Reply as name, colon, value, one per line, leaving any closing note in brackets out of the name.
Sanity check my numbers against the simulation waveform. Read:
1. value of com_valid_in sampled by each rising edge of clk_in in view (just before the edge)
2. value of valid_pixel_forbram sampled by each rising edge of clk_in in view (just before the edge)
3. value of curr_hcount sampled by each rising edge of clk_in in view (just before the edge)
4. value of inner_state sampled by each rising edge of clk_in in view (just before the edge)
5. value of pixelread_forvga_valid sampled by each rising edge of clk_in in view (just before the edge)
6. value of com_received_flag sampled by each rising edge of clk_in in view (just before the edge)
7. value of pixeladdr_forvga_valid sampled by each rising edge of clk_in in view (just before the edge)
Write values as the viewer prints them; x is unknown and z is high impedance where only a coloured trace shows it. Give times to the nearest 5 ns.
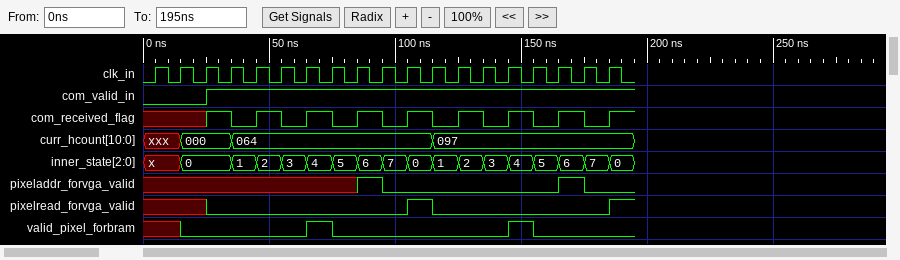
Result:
value of com_valid_in sampled by each rising edge of clk_in in view: 0 0 0 1 1 1 1 1 1 1 1 1 1 1 1 1 1 1 1
value of valid_pixel_forbram sampled by each rising edge of clk_in in view: x x 0 0 0 0 0 1 0 0 0 0 0 0 0 1 0 0 0
value of curr_hcount sampled by each rising edge of clk_in in view: xxx, xxx, 000, 000, 064, 064, 064, 064, 064, 064, 064, 064, 097, 097, 097, 097, 097, 097, 097
value of inner_state sampled by each rising edge of clk_in in view: x, x, 0, 0, 1, 2, 3, 4, 5, 6, 7, 0, 1, 2, 3, 4, 5, 6, 7
value of pixelread_forvga_valid sampled by each rising edge of clk_in in view: x x x 0 0 0 0 0 0 0 0 1 0 0 0 0 0 0 0
value of com_received_flag sampled by each rising edge of clk_in in view: x x x 1 0 1 0 1 0 1 0 1 0 1 0 1 0 1 0
value of pixeladdr_forvga_valid sampled by each rising edge of clk_in in view: x x x x x x x x x 1 0 0 0 0 0 0 0 1 0
